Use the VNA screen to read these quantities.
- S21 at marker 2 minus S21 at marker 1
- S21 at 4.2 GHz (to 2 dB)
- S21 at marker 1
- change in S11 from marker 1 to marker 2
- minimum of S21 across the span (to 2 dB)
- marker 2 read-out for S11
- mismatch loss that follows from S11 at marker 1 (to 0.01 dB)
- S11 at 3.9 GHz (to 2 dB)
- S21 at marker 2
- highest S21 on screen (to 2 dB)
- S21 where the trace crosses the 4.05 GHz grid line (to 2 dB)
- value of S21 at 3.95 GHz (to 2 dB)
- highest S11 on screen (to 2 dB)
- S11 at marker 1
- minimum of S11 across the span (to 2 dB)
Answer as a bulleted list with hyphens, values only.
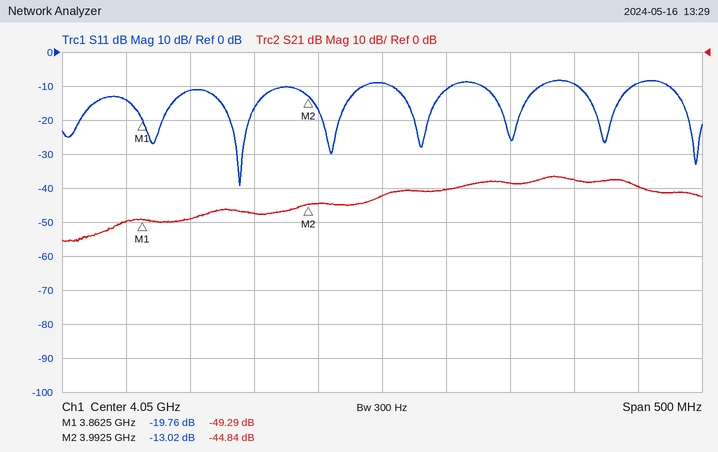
- 4.45 dB
- -38 dB
- -49.29 dB
- 6.74 dB
- -56 dB
- -13.02 dB
- 0.05 dB
- -12 dB
- -44.84 dB
- -36 dB
- -42 dB
- -48 dB
- -8 dB
- -19.76 dB
- -40 dB
